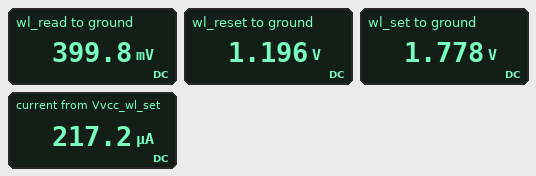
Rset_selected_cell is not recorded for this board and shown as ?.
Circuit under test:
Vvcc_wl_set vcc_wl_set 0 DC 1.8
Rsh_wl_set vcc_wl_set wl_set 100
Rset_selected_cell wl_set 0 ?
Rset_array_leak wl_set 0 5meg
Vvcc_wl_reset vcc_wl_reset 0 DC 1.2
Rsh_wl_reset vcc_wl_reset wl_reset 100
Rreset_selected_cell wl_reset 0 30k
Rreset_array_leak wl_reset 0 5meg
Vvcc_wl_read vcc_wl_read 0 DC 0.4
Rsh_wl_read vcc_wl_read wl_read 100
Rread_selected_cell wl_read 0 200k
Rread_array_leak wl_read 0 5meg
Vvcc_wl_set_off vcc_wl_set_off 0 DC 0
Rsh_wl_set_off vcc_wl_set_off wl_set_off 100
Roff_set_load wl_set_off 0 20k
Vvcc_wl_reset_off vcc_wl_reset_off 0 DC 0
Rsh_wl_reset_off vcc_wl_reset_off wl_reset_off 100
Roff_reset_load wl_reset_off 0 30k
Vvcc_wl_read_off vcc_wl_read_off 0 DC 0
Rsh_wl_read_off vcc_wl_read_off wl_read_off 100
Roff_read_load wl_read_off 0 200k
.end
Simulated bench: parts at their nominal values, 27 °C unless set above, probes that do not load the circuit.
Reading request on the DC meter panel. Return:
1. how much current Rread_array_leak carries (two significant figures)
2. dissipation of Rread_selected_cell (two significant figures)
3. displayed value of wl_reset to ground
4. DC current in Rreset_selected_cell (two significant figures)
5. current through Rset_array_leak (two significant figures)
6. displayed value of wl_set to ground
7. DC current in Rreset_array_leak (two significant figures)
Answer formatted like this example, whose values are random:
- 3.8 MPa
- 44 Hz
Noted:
- 80 nA
- 800 nW
- 1.196 V
- 40 µA
- 360 nA
- 1.778 V
- 240 nA
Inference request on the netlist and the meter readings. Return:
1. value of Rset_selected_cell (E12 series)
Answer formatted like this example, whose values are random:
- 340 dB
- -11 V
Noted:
- 8.2 kΩ
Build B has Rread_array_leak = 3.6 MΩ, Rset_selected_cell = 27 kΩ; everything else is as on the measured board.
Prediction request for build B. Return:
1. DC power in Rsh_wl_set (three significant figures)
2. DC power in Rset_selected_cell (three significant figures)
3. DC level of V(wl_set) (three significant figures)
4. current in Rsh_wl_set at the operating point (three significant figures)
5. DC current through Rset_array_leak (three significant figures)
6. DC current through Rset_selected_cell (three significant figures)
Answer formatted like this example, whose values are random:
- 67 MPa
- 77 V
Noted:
- 446 nW
- 119 µW
- 1.79 V
- 66.8 µA
- 359 nA
- 66.4 µA
